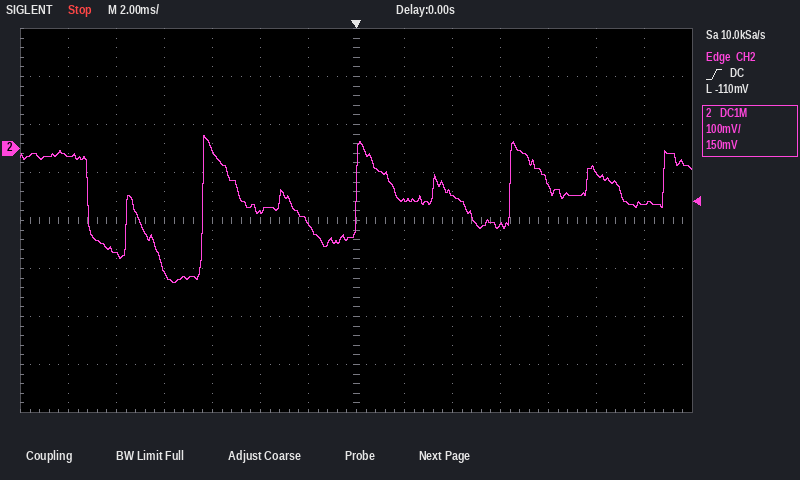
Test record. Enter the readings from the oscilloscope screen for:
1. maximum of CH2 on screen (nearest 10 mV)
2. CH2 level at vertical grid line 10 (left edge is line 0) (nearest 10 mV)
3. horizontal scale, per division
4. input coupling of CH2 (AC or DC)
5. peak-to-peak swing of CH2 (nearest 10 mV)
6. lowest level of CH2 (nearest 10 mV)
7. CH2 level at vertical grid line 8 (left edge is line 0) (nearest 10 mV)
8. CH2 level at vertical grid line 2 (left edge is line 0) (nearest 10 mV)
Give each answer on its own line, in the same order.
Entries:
30 mV
-160 mV
2 ms
DC
310 mV
-280 mV
-110 mV
-220 mV
